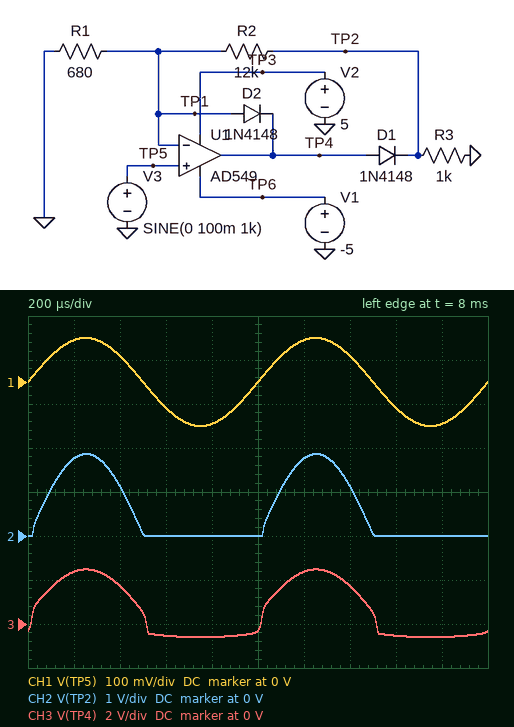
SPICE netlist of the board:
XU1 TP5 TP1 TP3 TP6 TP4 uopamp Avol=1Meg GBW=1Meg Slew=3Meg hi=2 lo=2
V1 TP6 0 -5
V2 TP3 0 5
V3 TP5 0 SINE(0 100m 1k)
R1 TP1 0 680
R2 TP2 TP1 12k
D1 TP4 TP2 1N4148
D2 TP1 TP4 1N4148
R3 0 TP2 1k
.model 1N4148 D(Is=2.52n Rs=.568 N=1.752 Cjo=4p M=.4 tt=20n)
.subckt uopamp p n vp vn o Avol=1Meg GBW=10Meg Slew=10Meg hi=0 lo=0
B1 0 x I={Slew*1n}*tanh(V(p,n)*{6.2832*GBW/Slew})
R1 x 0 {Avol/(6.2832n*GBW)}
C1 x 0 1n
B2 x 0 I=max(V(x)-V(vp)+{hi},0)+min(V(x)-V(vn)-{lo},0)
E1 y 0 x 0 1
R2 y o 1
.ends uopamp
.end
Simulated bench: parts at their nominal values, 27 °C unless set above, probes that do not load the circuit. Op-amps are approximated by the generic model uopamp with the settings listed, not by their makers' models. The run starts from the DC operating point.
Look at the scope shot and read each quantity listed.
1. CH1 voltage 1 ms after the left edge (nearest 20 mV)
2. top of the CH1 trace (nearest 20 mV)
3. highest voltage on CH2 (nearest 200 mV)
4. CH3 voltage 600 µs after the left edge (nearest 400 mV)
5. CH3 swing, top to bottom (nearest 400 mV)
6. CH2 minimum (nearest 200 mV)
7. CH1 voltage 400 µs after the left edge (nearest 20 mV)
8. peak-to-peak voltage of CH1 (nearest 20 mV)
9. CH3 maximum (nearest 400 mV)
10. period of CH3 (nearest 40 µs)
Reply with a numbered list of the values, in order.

1. 0 V
2. 100 mV
3. 1.8 V
4. -400 mV
5. 3.2 V
6. 0 V
7. 60 mV
8. 200 mV
9. 2.4 V
10. 1.00 ms
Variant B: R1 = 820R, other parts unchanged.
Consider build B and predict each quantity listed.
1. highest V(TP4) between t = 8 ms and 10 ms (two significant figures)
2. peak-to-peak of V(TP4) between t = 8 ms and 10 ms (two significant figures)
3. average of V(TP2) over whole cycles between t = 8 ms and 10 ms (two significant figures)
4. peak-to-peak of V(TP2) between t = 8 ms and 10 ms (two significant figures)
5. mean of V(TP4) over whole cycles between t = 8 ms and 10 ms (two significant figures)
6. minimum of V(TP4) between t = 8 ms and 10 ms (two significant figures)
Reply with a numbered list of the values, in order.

1. 2.2 V
2. 2.8 V
3. 490 mV
4. 1.6 V
5. 520 mV
6. -590 mV
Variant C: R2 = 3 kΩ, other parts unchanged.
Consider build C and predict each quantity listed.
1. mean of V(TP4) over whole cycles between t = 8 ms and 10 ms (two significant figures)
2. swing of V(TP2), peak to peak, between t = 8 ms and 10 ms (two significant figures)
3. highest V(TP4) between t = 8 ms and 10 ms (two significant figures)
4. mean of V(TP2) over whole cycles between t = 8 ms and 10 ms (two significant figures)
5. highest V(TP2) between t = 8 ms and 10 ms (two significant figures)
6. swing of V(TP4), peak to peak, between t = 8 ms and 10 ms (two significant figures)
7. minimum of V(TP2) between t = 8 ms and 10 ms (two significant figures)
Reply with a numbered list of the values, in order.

1. 170 mV
2. 570 mV
3. 1.1 V
4. 160 mV
5. 540 mV
6. 1.7 V
7. -25 mV
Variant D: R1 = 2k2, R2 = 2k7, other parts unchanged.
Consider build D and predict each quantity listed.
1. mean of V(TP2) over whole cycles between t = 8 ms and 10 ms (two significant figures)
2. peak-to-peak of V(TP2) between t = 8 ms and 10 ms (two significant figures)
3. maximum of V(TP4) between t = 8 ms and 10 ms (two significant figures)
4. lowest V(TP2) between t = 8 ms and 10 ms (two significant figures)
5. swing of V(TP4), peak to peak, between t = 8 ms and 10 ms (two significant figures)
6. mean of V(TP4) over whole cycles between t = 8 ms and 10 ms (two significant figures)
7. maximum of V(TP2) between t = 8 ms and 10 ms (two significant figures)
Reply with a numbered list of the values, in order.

1. 62 mV
2. 250 mV
3. 750 mV
4. -27 mV
5. 1.3 V
6. 69 mV
7. 220 mV
